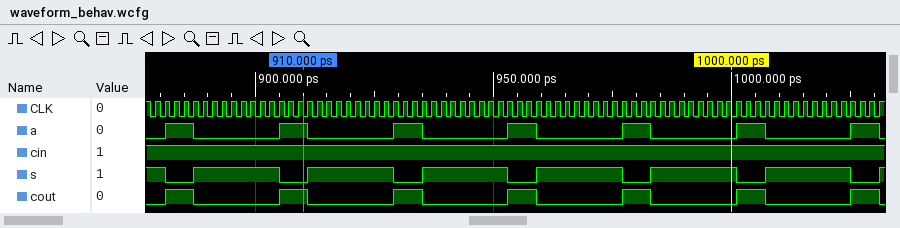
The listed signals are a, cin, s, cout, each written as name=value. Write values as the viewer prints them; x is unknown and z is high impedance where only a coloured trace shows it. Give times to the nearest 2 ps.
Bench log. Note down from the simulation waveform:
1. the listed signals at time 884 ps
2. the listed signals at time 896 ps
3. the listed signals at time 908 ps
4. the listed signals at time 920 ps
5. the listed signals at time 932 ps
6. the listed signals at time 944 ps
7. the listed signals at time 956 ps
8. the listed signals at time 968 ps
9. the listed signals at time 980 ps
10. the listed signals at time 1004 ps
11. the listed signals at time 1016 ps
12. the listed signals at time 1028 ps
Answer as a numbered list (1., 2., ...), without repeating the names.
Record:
1. a=1, cin=1, s=0, cout=1
2. a=0, cin=1, s=1, cout=0
3. a=1, cin=1, s=0, cout=1
4. a=0, cin=1, s=1, cout=0
5. a=1, cin=1, s=0, cout=1
6. a=0, cin=1, s=1, cout=0
7. a=1, cin=1, s=0, cout=1
8. a=0, cin=1, s=1, cout=0
9. a=1, cin=1, s=0, cout=1
10. a=1, cin=1, s=0, cout=1
11. a=0, cin=1, s=1, cout=0
12. a=1, cin=1, s=0, cout=1
